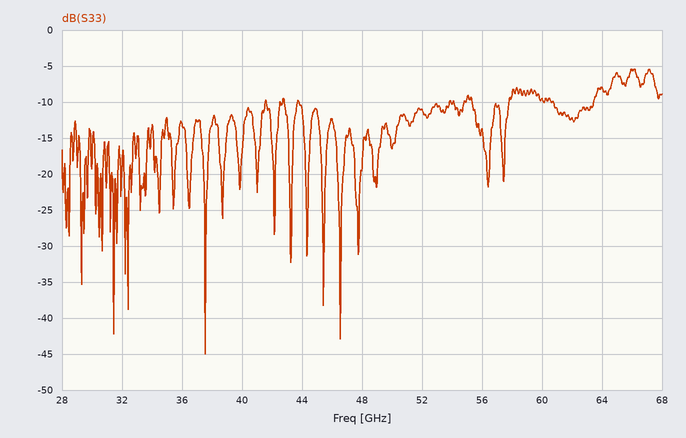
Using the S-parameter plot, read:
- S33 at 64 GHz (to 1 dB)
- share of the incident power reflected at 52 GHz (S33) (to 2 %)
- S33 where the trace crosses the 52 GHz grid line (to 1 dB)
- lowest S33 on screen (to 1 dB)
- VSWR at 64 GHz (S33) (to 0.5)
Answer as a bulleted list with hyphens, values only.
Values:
- -8 dB
- 8 %
- -11 dB
- -45 dB
- 2.5
